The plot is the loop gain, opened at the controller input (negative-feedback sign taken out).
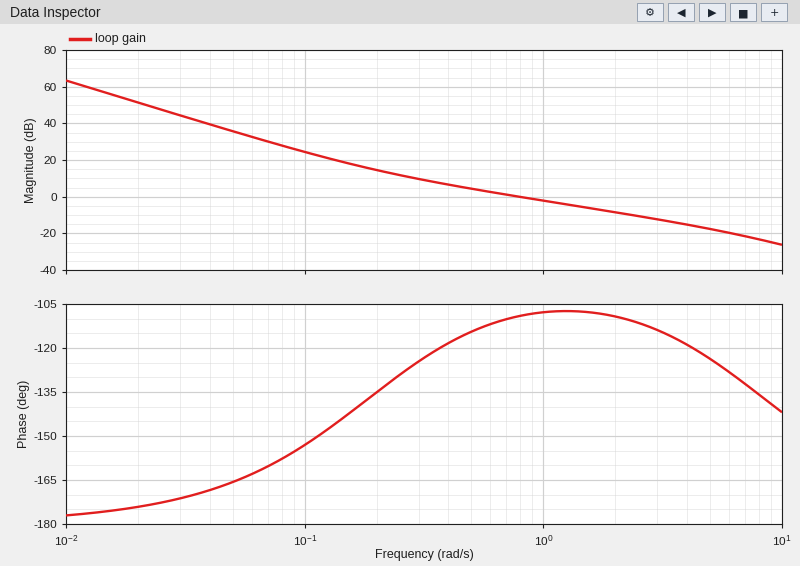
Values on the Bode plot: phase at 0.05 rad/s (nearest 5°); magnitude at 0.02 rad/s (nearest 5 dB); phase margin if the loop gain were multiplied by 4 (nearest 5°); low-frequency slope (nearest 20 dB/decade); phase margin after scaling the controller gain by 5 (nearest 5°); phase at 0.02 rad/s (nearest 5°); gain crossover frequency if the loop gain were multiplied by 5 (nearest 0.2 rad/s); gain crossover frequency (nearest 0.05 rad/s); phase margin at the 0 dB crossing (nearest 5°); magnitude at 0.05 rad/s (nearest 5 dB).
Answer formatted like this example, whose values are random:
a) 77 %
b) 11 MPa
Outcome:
a) -165°
b) 50 dB
c) 65°
d) -40 dB/decade
e) 65°
f) -175°
g) 3.6 rad/s
h) 0.80 rad/s
i) 70°
j) 35 dB
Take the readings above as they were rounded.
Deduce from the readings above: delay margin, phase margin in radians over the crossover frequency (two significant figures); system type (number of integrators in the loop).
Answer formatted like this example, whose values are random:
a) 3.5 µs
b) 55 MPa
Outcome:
a) 1.5 s
b) 2
